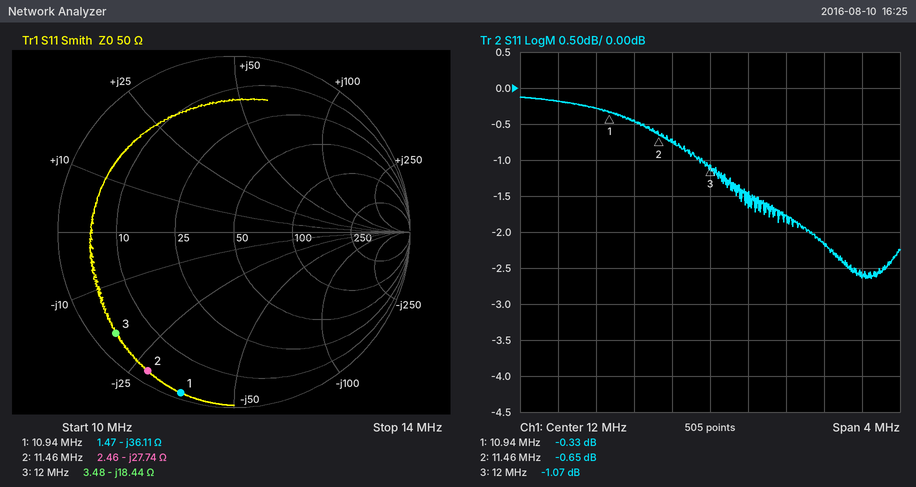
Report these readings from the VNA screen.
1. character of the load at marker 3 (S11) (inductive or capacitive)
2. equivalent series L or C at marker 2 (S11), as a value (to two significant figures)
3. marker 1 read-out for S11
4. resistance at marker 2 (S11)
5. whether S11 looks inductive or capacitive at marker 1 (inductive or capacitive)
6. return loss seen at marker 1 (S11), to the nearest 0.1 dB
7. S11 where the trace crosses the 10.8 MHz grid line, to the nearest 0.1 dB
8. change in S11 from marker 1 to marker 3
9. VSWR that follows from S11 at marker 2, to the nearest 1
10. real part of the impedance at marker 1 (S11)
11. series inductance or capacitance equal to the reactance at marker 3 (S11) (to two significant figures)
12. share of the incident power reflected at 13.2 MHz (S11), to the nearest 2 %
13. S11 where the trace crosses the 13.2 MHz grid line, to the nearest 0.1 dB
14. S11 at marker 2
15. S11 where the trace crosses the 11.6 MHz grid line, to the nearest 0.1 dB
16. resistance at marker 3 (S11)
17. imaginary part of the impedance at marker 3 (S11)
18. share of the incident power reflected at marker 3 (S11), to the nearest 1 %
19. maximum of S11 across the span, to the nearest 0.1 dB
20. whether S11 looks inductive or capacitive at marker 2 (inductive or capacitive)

capacitive
500 pF
-0.33 dB
2.46 Ω
capacitive
0.3 dB
-0.3 dB
-0.74 dB
27
1.47 Ω
720 pF
60 %
-2.2 dB
-0.65 dB
-0.7 dB
3.48 Ω
-18.44 Ω
78 %
-0.1 dB
capacitive
